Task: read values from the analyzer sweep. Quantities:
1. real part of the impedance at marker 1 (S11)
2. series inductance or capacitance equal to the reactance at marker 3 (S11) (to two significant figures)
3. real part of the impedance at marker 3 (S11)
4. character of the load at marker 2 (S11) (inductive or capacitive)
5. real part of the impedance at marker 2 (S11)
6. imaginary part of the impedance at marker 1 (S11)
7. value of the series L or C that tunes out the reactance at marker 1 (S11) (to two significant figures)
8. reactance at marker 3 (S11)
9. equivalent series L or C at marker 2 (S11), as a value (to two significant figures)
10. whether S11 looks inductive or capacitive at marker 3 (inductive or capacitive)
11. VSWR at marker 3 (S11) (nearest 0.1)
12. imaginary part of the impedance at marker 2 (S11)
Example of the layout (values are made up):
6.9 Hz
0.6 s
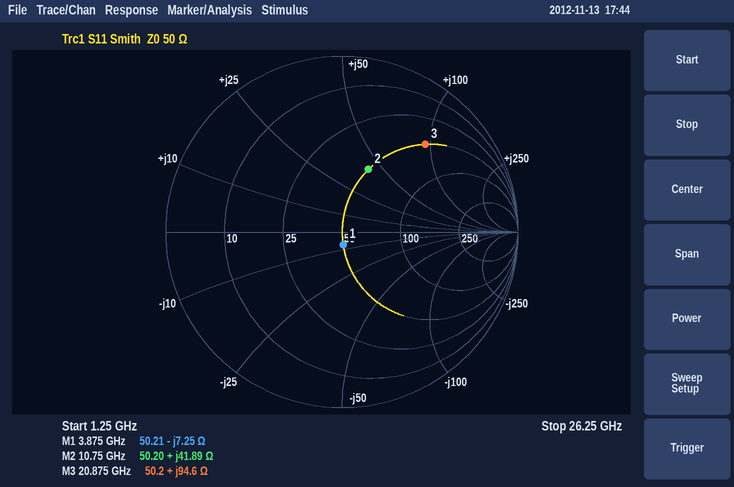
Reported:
50.21 Ω
720 pH
50.2 Ω
inductive
50.20 Ω
-7.25 Ω
300 pH
+94.6 Ω
620 pH
inductive
5.4
+41.89 Ω
